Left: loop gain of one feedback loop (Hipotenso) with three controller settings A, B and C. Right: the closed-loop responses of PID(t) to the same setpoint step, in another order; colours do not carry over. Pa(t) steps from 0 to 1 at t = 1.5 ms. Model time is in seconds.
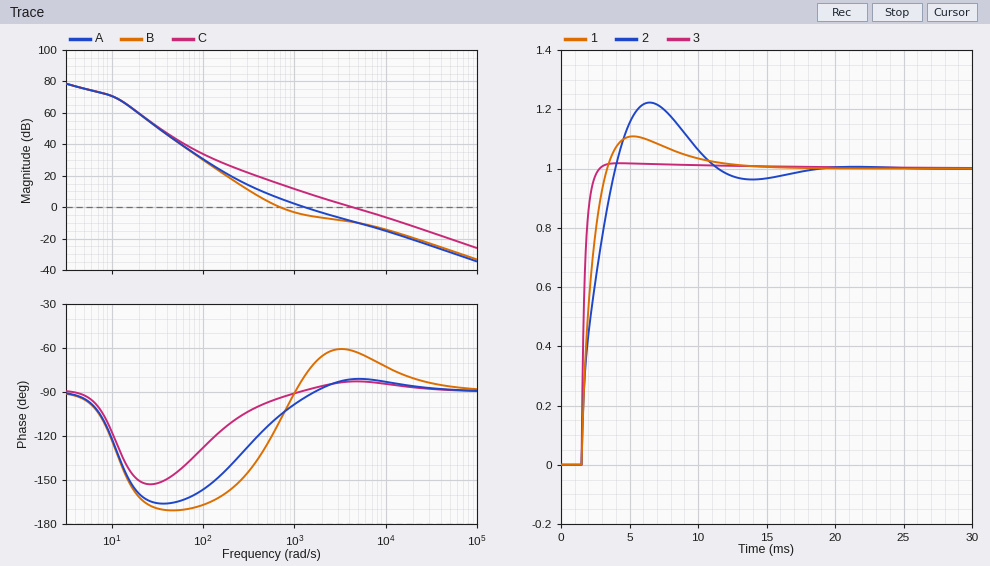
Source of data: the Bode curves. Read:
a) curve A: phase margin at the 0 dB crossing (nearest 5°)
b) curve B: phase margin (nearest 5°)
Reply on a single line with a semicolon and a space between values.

85°; 70°
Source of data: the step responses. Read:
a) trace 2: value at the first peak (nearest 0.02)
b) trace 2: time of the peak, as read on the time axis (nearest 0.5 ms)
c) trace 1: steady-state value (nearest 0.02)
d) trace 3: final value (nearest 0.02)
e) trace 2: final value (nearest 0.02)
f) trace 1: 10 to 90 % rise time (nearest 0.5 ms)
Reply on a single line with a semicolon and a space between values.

1.22; 6.5 ms; 1.00; 1.00; 1.00; 1.5 ms
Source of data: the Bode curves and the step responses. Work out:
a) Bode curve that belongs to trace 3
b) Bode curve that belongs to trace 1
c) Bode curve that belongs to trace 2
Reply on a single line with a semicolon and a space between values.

C; A; B
